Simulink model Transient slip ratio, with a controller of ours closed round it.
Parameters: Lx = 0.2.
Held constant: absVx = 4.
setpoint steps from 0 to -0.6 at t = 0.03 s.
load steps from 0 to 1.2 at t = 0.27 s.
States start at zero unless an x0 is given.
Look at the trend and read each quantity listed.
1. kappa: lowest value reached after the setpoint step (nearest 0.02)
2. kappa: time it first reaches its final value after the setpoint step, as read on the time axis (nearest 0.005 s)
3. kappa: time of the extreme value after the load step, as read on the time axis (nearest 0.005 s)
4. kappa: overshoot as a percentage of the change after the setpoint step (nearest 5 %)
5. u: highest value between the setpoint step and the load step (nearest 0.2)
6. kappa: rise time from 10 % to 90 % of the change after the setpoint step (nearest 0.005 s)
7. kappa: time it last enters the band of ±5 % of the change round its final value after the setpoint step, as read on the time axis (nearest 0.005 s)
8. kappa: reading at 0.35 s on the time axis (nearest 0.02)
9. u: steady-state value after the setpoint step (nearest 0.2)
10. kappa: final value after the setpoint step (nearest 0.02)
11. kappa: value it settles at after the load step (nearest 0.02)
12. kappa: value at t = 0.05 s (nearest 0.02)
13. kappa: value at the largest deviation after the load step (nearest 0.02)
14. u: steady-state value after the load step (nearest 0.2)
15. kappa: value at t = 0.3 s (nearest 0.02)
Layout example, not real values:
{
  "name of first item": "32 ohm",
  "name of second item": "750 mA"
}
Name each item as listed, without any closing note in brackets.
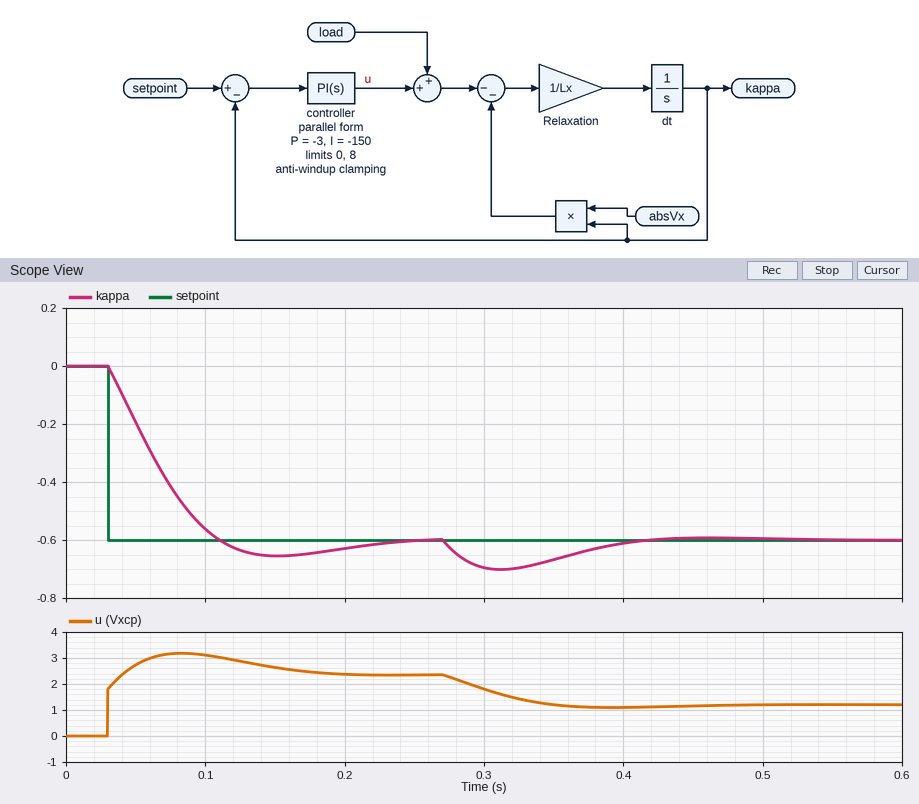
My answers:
{
  "kappa: lowest value reached after the setpoint step": "-0.66",
  "kappa: time it first reaches its final value after the setpoint step, as read on the time axis": "0.110 s",
  "kappa: time of the extreme value after the load step, as read on the time axis": "0.310 s",
  "kappa: overshoot as a percentage of the change after the setpoint step": "10 %",
  "u: highest value between the setpoint step and the load step": "3.2",
  "kappa: rise time from 10 % to 90 % of the change after the setpoint step": "0.060 s",
  "kappa: time it last enters the band of ±5 % of the change round its final value after the setpoint step, as read on the time axis": "0.200 s",
  "kappa: reading at 0.35 s on the time axis": "-0.66",
  "u: steady-state value after the setpoint step": "2.4",
  "kappa: final value after the setpoint step": "-0.60",
  "kappa: value it settles at after the load step": "-0.60",
  "kappa: value at t = 0.05 s": "-0.20",
  "kappa: value at the largest deviation after the load step": "-0.70",
  "u: steady-state value after the load step": "1.2",
  "kappa: value at t = 0.3 s": "-0.70"
}
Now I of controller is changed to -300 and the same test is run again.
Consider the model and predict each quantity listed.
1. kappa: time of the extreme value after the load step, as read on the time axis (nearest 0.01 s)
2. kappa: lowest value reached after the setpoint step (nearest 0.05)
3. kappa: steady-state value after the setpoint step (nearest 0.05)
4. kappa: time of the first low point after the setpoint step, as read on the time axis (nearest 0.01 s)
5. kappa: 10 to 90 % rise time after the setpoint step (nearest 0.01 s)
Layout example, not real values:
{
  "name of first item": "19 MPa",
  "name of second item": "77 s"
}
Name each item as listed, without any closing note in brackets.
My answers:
{
  "kappa: time of the extreme value after the load step, as read on the time axis": "0.30 s",
  "kappa: lowest value reached after the setpoint step": "-0.75",
  "kappa: steady-state value after the setpoint step": "-0.60",
  "kappa: time of the first low point after the setpoint step, as read on the time axis": "0.11 s",
  "kappa: 10 to 90 % rise time after the setpoint step": "0.04 s"
}
